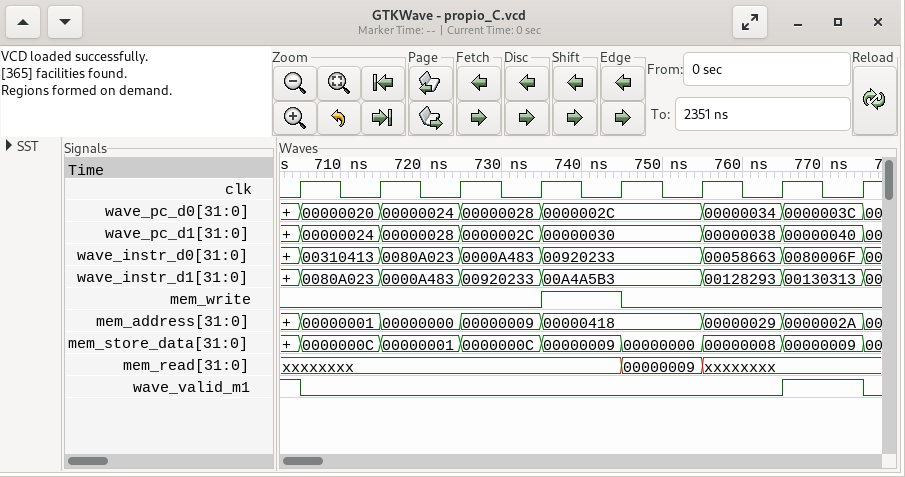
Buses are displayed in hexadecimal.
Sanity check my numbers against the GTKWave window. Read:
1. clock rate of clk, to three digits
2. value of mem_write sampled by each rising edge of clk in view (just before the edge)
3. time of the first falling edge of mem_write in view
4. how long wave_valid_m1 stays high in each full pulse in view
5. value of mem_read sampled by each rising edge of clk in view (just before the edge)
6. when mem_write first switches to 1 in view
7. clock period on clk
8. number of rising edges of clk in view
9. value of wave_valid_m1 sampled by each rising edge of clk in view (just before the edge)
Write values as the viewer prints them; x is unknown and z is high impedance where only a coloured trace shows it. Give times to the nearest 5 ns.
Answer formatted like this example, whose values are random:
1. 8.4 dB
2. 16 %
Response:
1. 100 MHz
2. 0 0 0 0 1 0 0 0
3. 745 ns
4. 10 ns
5. xxxxxxxx, xxxxxxxx, xxxxxxxx, xxxxxxxx, xxxxxxxx, 00000009, xxxxxxxx, xxxxxxxx
6. 735 ns
7. 10 ns
8. 8
9. 1 0 0 0 0 0 0 1
